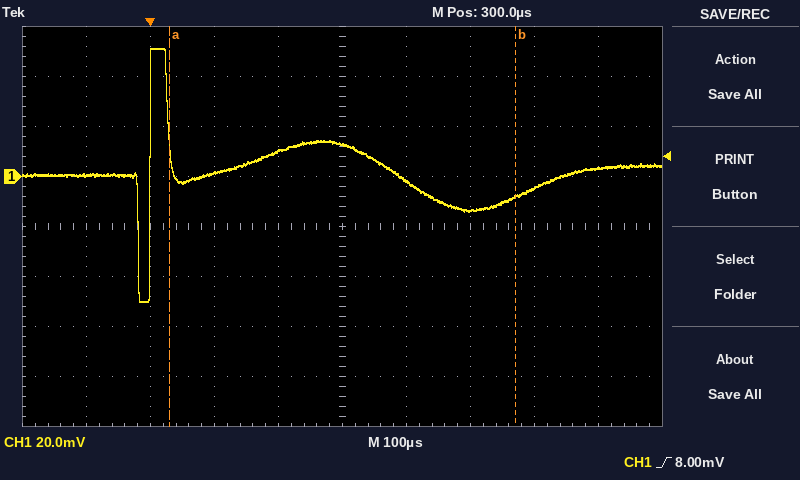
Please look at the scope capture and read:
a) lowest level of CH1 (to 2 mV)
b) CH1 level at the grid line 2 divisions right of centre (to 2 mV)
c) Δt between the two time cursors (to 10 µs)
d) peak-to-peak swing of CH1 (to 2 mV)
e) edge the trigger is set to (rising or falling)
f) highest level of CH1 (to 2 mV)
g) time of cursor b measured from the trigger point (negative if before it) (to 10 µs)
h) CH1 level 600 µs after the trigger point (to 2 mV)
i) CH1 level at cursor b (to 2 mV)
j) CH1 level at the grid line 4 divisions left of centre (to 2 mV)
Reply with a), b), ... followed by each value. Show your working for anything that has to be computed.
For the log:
a) -50 mV
b) -14 mV
c) 540 µs
d) 52 mV − (-50 mV) = 102 mV
e) rising
f) 52 mV
g) +570 µs
h) -4 mV
i) -8 mV
j) 0 mV
